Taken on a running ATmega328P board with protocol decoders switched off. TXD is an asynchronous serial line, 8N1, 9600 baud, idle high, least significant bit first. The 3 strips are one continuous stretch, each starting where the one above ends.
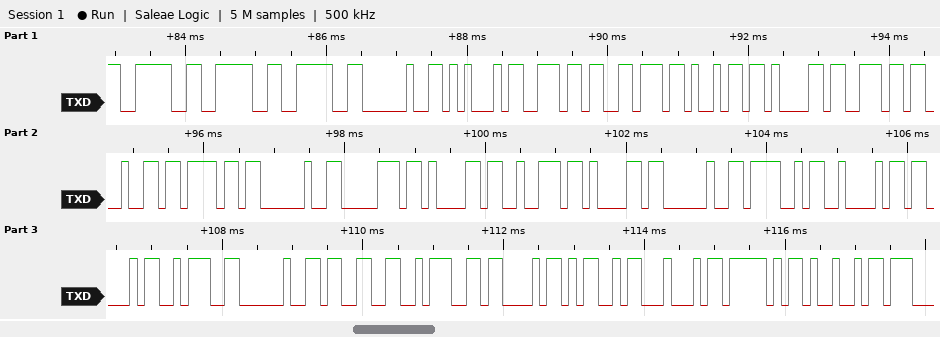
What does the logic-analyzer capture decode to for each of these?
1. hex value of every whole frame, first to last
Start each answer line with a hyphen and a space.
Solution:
- 3E 3E 3E 20 45 6E 76 69 61 6E 64 6F 20 70 61 72 61 20 4F 42 43 3A 20 33 3A 43 4D 44 5F 49
